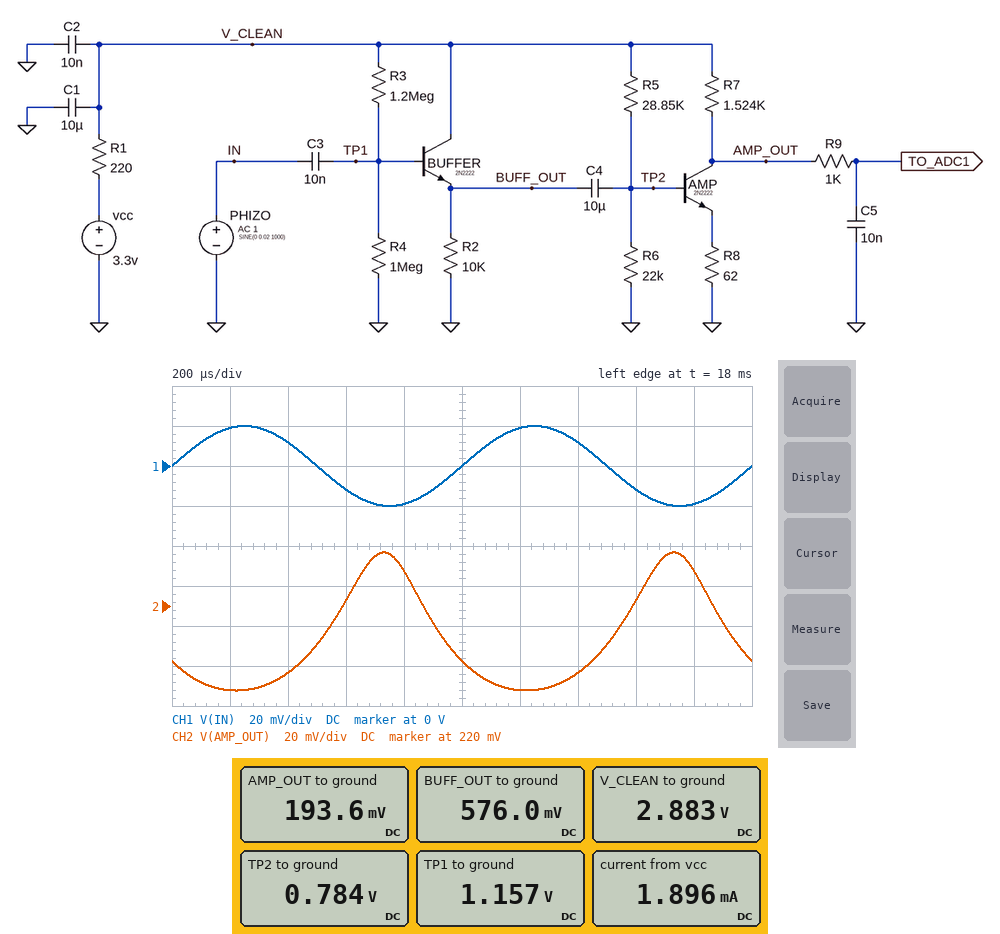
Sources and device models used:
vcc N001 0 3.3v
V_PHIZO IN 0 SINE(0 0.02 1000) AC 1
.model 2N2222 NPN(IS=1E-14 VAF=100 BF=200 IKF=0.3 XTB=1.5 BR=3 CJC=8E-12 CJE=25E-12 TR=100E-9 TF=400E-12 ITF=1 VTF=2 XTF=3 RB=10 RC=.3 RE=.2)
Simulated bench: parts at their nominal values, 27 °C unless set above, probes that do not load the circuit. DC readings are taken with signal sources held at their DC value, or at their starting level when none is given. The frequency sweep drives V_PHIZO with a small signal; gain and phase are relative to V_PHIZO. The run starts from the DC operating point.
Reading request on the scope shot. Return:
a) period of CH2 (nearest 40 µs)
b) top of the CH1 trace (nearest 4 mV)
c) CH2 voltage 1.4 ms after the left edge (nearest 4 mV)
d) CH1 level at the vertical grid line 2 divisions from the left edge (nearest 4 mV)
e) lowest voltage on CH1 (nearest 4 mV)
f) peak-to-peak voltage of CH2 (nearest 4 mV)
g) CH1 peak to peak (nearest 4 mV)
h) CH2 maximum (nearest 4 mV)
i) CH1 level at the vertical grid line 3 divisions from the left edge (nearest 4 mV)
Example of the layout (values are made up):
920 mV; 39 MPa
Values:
1.00 ms; 20 mV; 188 mV; 12 mV; -20 mV; 68 mV; 40 mV; 248 mV; -12 mV
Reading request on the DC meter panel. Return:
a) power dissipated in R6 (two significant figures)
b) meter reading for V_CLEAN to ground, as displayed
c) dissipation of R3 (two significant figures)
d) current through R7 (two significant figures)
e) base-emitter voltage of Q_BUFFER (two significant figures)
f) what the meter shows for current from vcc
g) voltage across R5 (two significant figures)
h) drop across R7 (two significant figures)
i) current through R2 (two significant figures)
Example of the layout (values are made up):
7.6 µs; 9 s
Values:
28 µW; 2.883 V; 2.5 µW; 1.8 mA; 580 mV; 1.896 mA; 2.1 V; 2.7 V; 58 µA
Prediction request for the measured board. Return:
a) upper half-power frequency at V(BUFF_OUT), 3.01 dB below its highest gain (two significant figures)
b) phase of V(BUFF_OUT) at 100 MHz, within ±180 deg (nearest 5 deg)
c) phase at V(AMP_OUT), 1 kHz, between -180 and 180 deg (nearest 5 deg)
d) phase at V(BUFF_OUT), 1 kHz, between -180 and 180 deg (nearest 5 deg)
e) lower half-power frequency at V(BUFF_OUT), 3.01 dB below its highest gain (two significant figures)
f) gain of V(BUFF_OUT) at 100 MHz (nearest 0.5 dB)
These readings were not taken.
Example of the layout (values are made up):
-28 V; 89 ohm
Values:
3.4 GHz; 20 deg; -170 deg; 5 deg; 54 MHz; -2.5 dB
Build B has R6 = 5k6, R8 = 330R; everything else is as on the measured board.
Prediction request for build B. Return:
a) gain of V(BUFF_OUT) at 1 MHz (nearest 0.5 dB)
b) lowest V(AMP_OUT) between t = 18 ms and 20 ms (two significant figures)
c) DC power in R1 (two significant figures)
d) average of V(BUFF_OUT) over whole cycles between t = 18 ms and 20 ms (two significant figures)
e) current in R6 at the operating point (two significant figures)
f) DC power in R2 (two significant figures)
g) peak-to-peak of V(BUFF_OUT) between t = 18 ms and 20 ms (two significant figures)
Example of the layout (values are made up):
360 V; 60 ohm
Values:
-1.0 dB; 3.2 V; 6.7 µW; 710 mV; 95 µA; 50 µW; 36 mV
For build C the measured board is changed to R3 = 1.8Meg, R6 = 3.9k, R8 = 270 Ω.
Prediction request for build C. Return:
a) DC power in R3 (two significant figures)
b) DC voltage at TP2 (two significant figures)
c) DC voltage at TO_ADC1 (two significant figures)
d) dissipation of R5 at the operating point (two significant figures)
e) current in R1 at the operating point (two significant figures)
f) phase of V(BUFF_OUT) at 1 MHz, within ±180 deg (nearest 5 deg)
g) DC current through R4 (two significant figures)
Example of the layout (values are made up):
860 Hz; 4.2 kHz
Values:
2.8 µW; 390 mV; 3.3 V; 290 µW; 150 µA; -5 deg; 1.0 µA
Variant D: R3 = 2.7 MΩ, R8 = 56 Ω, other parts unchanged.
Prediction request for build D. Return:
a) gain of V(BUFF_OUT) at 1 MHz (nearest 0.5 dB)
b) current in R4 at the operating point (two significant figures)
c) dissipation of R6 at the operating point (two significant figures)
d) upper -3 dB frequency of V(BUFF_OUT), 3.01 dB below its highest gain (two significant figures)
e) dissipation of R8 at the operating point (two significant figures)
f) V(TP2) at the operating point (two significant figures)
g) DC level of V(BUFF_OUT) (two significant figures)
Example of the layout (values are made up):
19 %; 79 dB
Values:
-23.0 dB; 720 nA; 27 µW; 3.7 GHz; 180 µW; 770 mV; 170 mV
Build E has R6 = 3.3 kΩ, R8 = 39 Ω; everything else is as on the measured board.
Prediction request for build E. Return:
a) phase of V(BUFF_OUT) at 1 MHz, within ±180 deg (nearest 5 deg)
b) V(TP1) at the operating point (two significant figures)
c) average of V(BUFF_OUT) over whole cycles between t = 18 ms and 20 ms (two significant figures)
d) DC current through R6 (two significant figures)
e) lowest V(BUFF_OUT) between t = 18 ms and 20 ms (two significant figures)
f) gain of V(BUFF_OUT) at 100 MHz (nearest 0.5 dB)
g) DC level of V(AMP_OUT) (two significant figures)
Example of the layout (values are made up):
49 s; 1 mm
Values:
-5 deg; 1.3 V; 710 mV; 100 µA; 690 mV; -4.0 dB; 3.3 V
